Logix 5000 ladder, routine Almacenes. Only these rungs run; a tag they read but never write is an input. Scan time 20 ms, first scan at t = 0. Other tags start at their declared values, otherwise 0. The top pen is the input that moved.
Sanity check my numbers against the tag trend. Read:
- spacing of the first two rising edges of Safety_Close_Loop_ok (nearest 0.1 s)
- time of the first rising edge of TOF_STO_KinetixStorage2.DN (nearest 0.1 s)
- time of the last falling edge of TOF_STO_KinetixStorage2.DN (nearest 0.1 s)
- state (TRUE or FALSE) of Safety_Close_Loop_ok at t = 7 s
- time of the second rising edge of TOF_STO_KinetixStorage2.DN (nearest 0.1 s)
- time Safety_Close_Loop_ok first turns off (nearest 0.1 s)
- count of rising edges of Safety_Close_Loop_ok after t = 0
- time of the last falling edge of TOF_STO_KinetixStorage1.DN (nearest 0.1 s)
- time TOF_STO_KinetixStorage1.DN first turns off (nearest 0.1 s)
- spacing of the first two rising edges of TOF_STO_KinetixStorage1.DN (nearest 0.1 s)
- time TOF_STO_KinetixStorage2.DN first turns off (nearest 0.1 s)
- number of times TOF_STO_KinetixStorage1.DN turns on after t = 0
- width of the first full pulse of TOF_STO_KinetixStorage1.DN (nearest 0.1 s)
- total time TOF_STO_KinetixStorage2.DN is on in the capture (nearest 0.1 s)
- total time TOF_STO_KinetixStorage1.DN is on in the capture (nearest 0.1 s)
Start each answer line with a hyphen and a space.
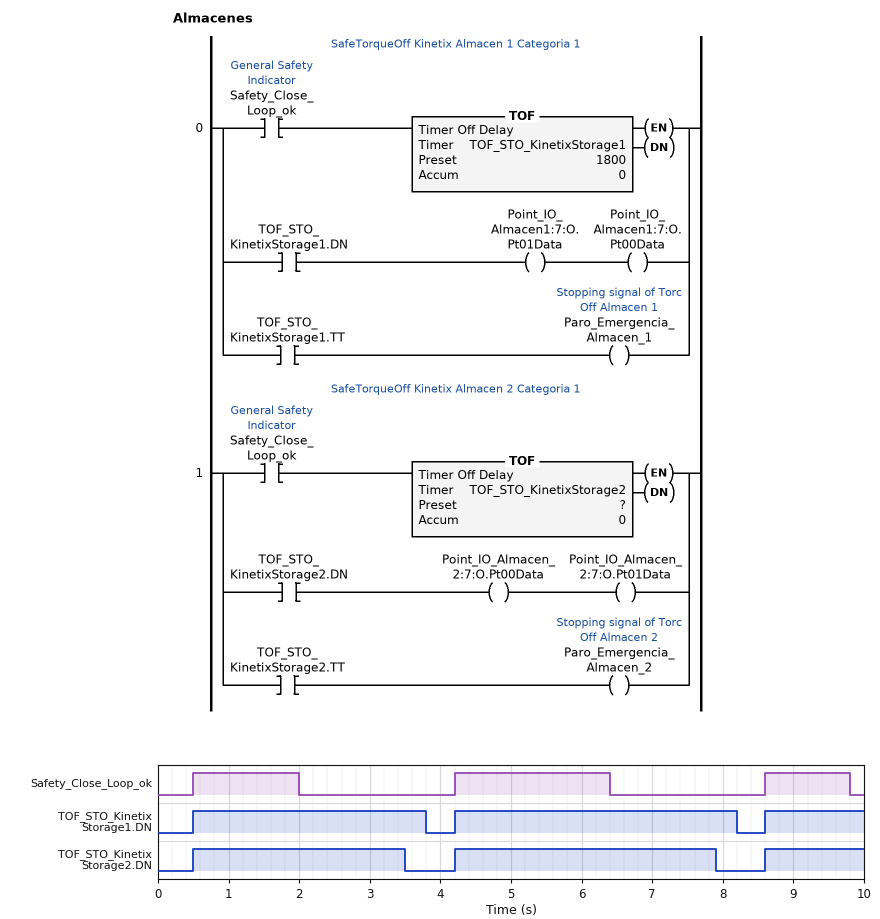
- 3.7 s
- 0.5 s
- 7.9 s
- FALSE
- 4.2 s
- 2.0 s
- 3
- 8.2 s
- 3.8 s
- 3.7 s
- 3.5 s
- 3
- 3.3 s
- 8.1 s
- 8.7 s
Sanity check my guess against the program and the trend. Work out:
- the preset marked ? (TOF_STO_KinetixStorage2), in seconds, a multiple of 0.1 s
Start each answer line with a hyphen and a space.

- 1.5 s
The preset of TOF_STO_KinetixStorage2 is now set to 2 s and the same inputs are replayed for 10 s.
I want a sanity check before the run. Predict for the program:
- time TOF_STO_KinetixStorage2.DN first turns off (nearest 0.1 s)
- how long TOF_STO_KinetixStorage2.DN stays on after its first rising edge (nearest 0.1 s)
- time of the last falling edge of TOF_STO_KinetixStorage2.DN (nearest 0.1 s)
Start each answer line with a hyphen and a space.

- 4.0 s
- 3.5 s
- 8.4 s
